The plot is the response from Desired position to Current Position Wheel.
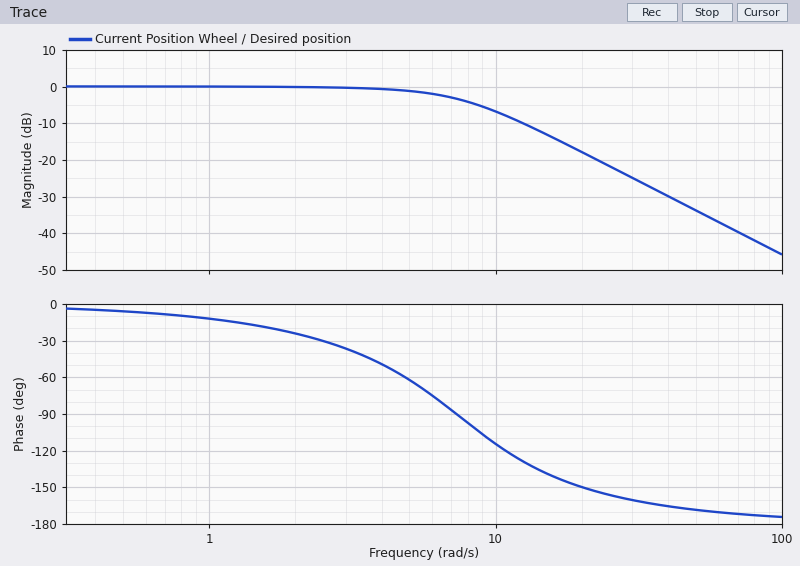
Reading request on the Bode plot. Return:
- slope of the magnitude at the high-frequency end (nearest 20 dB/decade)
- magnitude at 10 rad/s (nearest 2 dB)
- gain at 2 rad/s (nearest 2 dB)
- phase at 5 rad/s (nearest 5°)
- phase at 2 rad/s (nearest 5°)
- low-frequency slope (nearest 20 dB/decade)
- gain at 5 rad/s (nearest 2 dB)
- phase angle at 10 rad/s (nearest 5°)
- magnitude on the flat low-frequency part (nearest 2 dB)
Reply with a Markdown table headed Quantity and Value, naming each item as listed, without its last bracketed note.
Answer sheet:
| Quantity | Value |
|---|---|
| slope of the magnitude at the high-frequency end | -40 dB/decade |
| magnitude at 10 rad/s | -6 dB |
| gain at 2 rad/s | 0 dB |
| phase at 5 rad/s | -60° |
| phase at 2 rad/s | -25° |
| low-frequency slope | 0 dB/decade |
| gain at 5 rad/s | -2 dB |
| phase angle at 10 rad/s | -115° |
| magnitude on the flat low-frequency part | 0 dB |
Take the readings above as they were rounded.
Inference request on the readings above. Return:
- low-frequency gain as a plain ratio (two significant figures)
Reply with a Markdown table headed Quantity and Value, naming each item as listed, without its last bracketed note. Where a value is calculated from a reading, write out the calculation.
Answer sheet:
| Quantity | Value |
|---|---|
| low-frequency gain as a plain ratio | 10^(0 / 20) = 1.0 |
